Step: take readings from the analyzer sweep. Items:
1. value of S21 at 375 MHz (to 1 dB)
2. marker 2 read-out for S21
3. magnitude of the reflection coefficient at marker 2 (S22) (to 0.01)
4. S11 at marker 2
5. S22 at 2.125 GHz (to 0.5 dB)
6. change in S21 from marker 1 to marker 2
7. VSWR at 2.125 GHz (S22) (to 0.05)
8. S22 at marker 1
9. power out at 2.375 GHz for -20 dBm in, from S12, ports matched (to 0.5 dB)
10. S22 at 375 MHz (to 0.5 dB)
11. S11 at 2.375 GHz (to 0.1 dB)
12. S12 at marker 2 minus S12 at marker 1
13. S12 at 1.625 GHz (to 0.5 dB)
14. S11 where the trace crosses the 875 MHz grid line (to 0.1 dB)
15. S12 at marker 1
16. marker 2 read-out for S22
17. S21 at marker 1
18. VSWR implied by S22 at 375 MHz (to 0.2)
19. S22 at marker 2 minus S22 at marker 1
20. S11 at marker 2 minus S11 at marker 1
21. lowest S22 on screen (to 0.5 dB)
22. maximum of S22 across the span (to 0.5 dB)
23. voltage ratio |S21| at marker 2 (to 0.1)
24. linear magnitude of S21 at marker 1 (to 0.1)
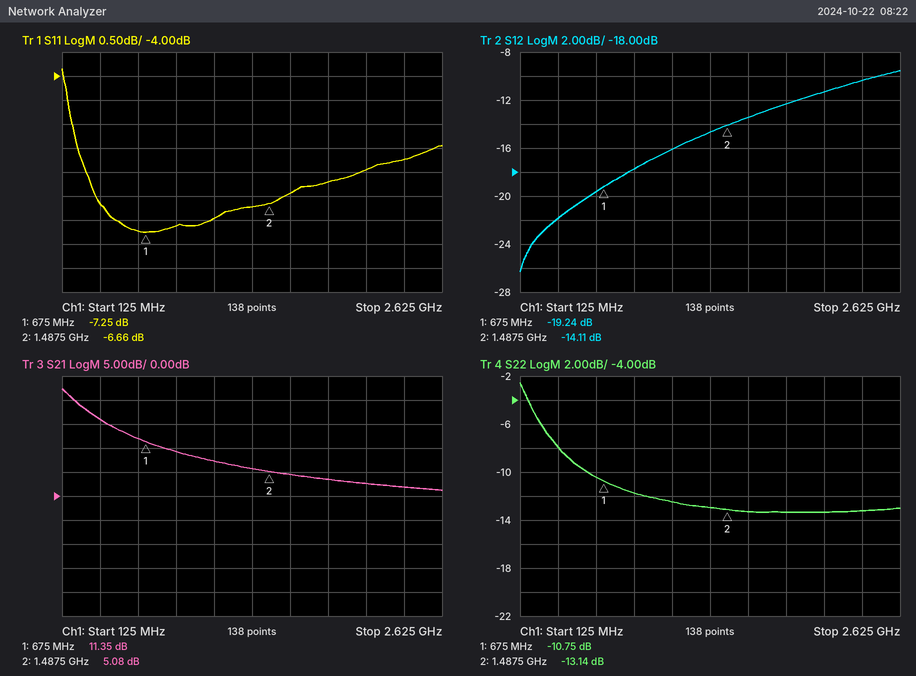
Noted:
16 dB
5.08 dB
0.22
-6.66 dB
-13.5 dB
-6.27 dB
1.55
-10.75 dB
-30.5 dBm
-8.0 dB
-5.7 dB
5.13 dB
-13.5 dB
-7.1 dB
-19.24 dB
-13.14 dB
11.35 dB
2.4
-2.39 dB
0.59 dB
-13.5 dB
-2.5 dB
1.8
3.7
